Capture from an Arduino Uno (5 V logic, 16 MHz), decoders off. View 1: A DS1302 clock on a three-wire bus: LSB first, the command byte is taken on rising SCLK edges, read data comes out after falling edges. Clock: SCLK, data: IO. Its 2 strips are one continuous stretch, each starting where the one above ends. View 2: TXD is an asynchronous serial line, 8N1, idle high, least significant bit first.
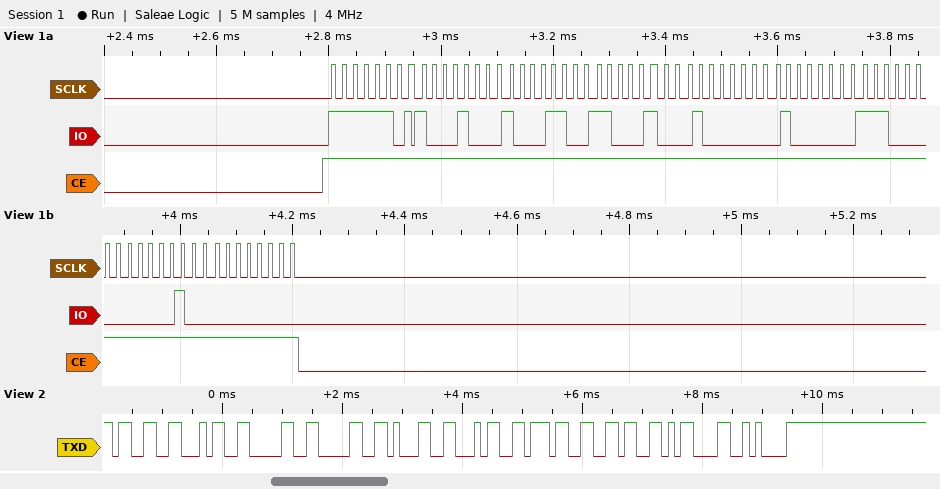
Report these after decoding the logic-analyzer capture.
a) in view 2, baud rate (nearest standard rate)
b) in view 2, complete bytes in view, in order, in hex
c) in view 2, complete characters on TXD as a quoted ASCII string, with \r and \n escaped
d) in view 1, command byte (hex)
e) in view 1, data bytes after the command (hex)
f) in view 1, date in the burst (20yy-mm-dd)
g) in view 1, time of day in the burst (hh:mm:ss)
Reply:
9600 baud
33 34 30 30 31 34 37 36 0D 0A
"34001476\r\n"
0xBF
11 31 23 02 02 07 20 00
2020-02-02
23:31:11
